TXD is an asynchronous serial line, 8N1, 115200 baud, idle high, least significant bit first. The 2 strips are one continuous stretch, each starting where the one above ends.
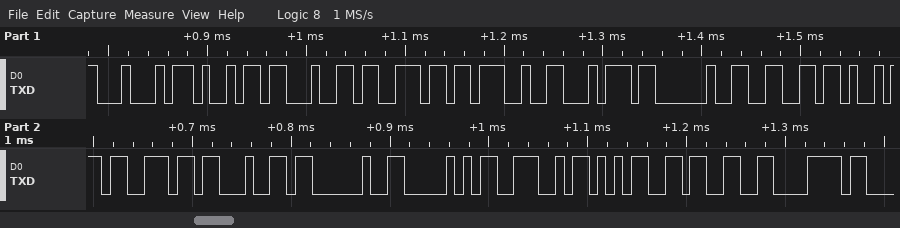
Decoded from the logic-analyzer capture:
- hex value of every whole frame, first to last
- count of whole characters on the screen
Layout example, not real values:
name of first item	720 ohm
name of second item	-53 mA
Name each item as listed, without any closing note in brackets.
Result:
hex value of every whole frame, first to last	44 69 64 6E 27 74 20 66 69 6E 64 20 50 4E 35 33 78
count of whole characters on the screen	17
